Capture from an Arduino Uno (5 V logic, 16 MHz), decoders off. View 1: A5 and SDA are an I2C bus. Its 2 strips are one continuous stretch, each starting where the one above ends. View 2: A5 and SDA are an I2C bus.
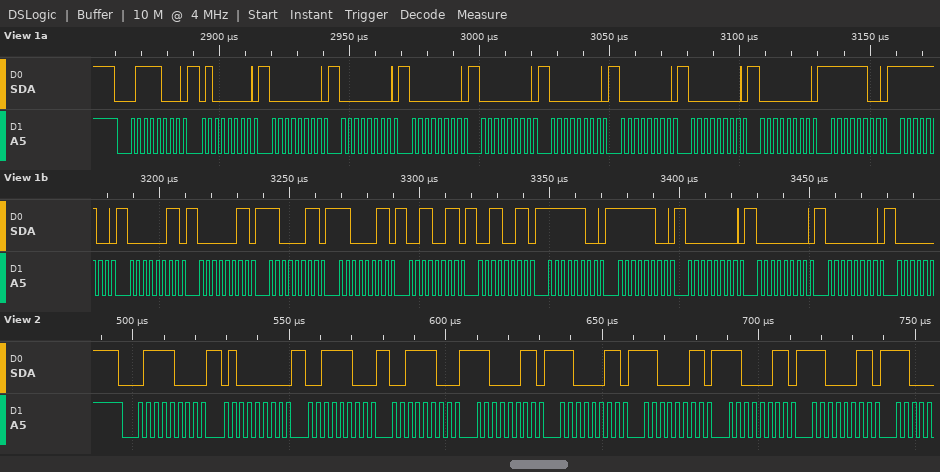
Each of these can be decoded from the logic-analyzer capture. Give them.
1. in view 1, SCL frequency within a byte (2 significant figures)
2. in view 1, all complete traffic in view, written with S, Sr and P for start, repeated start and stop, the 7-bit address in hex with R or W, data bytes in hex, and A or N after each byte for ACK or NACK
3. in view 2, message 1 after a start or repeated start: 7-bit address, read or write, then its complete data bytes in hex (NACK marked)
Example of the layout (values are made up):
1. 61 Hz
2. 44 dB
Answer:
1. 400 kHz
2. S 3CW A 40 A 00 A 00 A 00 A 00 A 00 A 00 A 00 A 00 A FC A FC A 03 A 03 A C3 A C3 A 33 A 33 A FC A FC A 00 A 00 A 00 A
3. 0x3C write: 40 3C 3C C3 C3 C3 C3 C3
